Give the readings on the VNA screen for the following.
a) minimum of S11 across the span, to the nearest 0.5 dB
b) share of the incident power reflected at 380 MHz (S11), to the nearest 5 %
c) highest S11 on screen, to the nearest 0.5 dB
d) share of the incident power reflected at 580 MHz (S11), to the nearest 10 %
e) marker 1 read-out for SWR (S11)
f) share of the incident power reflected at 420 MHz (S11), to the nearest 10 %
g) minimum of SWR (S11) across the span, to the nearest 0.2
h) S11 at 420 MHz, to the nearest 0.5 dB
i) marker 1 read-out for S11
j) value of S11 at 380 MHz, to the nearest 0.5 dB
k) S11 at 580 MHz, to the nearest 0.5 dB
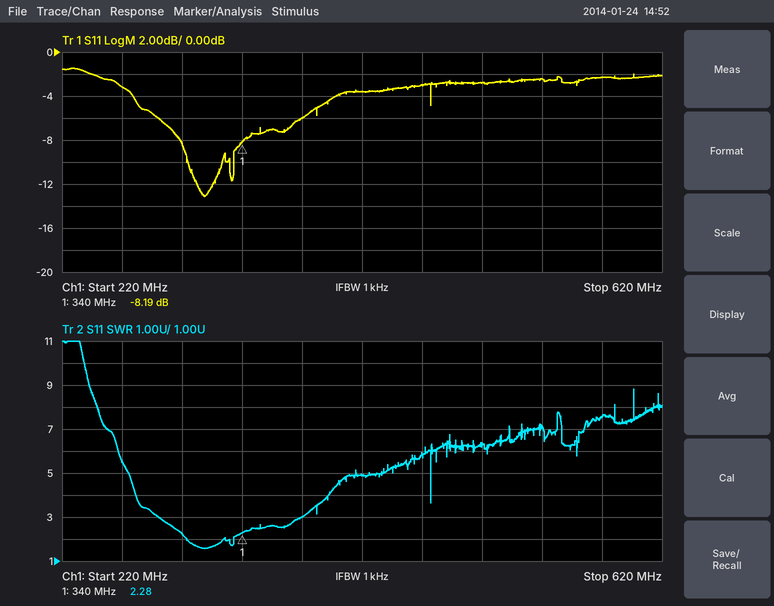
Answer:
-13.0 dB
25 %
-1.5 dB
60 %
2.28
40 %
1.6
-3.5 dB
-8.19 dB
-6.0 dB
-2.5 dB
